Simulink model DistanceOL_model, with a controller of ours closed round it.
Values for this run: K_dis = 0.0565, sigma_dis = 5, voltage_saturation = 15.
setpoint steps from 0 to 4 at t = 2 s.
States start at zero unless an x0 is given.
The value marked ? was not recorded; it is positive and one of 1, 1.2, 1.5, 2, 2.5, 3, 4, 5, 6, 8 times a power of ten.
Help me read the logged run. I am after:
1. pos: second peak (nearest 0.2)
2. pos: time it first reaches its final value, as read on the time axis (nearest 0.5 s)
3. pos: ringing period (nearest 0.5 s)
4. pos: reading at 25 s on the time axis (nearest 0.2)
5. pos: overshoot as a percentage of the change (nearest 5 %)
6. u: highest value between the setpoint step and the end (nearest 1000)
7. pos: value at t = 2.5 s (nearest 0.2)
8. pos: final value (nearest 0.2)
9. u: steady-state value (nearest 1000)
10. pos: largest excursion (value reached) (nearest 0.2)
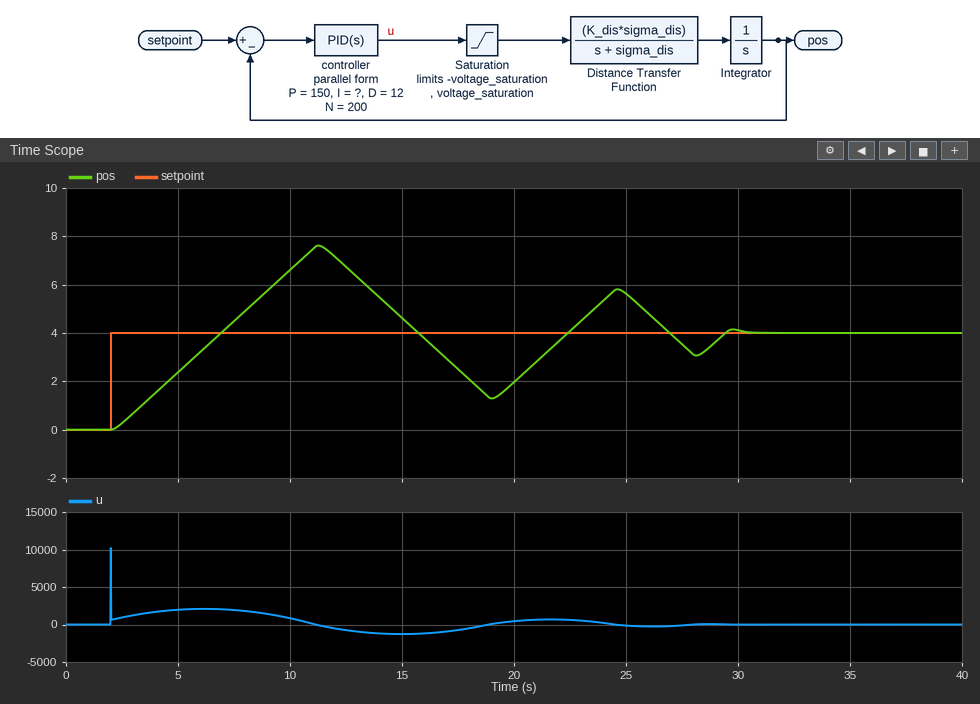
5.8
7.0 s
13.5 s
5.6
90 %
10000
0.2
4.0
0
7.6
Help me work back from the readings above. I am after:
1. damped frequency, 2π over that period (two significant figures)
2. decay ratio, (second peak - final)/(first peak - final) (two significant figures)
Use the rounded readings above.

0.47 rad/s
0.50
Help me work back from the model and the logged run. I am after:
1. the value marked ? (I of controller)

200
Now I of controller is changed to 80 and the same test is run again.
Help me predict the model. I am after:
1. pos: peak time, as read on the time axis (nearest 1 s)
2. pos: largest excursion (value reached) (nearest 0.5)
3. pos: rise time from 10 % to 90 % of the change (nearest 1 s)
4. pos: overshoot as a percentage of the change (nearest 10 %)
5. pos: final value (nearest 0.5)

10 s
7.0
4 s
70 %
4.0
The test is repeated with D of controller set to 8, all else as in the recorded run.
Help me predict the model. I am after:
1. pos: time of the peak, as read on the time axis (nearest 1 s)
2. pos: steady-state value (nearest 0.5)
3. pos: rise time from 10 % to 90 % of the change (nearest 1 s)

11 s
4.0
4 s
